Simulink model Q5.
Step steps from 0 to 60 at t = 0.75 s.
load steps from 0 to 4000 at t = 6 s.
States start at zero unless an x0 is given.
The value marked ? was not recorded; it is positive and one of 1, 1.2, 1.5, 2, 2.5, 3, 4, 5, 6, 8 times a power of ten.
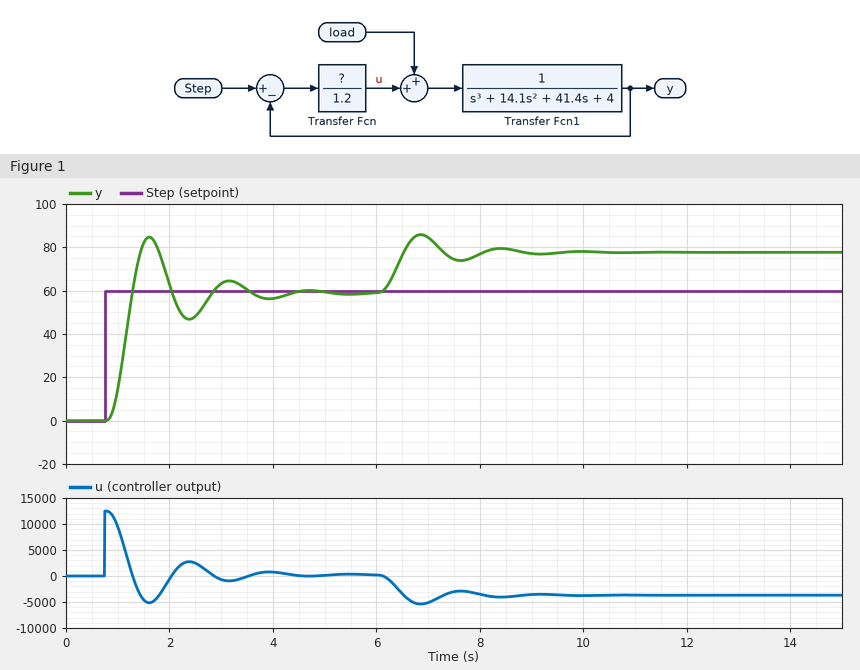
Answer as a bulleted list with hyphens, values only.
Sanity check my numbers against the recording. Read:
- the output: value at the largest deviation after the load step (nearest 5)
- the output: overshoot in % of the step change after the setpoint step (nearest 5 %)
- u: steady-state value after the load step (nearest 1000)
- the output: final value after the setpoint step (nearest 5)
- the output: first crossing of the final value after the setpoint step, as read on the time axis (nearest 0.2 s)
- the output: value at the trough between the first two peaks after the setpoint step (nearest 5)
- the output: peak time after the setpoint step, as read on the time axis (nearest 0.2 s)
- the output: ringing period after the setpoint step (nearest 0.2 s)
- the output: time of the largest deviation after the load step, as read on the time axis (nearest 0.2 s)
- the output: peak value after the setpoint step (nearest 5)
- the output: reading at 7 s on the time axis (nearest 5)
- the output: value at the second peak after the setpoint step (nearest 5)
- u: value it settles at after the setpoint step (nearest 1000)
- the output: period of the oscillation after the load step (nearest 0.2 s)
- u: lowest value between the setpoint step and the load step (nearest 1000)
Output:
- 85
- 45 %
- -4000
- 60
- 1.2 s
- 45
- 1.6 s
- 1.6 s
- 6.8 s
- 85
- 85
- 65
- 0
- 1.6 s
- -5000
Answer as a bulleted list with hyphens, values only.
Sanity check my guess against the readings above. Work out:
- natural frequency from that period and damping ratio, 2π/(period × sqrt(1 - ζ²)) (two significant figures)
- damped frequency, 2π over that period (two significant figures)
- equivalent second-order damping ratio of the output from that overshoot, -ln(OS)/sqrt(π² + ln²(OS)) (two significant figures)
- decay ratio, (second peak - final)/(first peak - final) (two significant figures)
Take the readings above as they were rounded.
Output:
- 4.1 rad/s
- 3.9 rad/s
- 0.25
- 0.20
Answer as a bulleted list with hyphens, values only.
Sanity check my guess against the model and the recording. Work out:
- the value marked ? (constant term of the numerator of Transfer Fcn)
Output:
- 250
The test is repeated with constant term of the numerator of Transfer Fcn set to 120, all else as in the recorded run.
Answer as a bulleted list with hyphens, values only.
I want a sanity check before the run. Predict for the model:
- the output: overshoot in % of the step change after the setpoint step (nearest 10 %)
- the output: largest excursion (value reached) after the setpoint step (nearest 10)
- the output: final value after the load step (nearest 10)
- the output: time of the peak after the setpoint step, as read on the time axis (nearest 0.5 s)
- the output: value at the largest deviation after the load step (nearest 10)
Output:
- 20 %
- 70
- 100
- 2.0 s
- 100
